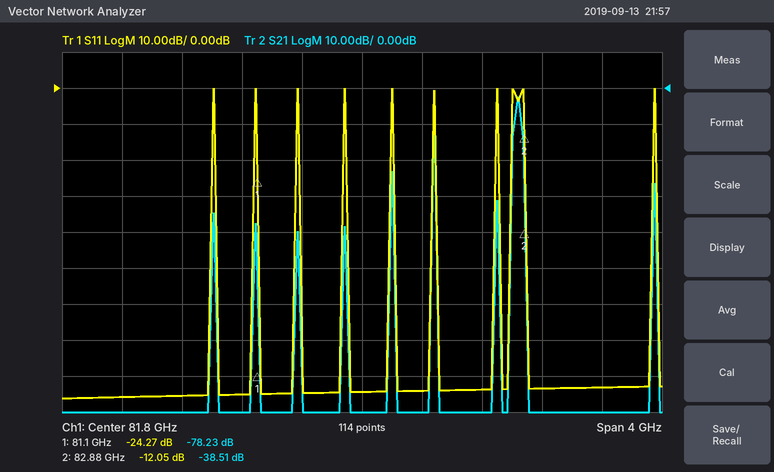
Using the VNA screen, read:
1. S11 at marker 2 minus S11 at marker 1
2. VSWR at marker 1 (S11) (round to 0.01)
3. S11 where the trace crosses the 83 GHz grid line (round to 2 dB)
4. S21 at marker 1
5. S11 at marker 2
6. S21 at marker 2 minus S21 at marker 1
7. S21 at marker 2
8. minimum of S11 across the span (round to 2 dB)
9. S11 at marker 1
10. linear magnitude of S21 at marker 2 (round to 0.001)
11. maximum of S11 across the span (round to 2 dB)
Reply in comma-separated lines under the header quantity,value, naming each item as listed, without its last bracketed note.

quantity,value
S11 at marker 2 minus S11 at marker 1,12.22 dB
VSWR at marker 1 (S11),1.13
S11 where the trace crosses the 83 GHz grid line,-84 dB
S21 at marker 1,-78.23 dB
S11 at marker 2,-12.05 dB
S21 at marker 2 minus S21 at marker 1,39.72 dB
S21 at marker 2,-38.51 dB
minimum of S11 across the span,-86 dB
S11 at marker 1,-24.27 dB
linear magnitude of S21 at marker 2,0.012
maximum of S11 across the span,0 dB
